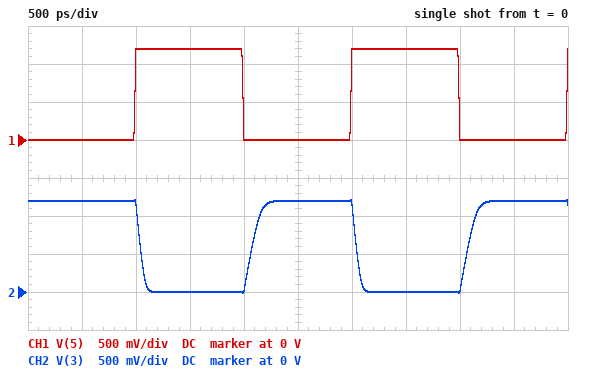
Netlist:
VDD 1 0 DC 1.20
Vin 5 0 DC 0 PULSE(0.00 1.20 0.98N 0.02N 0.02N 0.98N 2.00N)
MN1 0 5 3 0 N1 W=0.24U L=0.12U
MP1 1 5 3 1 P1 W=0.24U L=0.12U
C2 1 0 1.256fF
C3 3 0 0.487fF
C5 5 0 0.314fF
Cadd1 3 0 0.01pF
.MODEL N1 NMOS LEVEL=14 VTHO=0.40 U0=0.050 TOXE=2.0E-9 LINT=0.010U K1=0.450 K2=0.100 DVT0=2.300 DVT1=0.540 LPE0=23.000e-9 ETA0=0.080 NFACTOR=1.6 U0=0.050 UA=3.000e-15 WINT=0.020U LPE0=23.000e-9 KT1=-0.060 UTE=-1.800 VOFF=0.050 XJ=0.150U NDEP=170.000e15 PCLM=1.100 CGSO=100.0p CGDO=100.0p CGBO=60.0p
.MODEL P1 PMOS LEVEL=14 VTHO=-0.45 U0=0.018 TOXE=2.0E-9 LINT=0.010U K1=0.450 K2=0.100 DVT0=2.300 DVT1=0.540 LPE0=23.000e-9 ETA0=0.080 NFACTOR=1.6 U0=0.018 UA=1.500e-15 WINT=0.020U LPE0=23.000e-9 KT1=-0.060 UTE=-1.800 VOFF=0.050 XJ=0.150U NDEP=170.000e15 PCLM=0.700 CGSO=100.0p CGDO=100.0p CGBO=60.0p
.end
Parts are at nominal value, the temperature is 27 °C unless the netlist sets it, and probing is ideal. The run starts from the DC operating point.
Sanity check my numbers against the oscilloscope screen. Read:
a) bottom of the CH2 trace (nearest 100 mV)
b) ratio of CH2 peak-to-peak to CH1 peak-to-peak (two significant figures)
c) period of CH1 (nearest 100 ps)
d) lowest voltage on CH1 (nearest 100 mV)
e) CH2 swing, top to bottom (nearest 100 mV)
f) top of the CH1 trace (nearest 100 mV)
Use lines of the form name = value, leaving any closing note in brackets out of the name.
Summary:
bottom of the CH2 trace = 0 V
ratio of CH2 peak-to-peak to CH1 peak-to-peak = 1.0
period of CH1 = 2.0 ns
lowest voltage on CH1 = 0 V
CH2 swing, top to bottom = 1.2 V
top of the CH1 trace = 1.2 V
